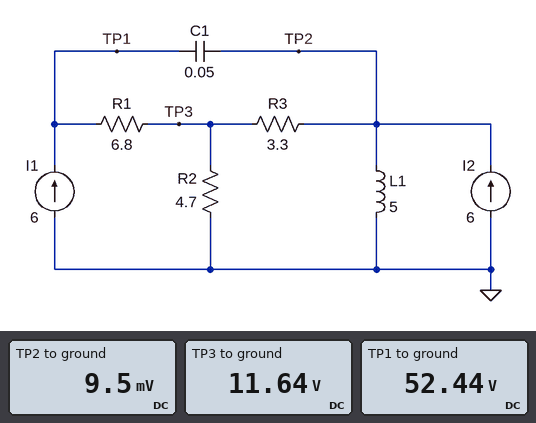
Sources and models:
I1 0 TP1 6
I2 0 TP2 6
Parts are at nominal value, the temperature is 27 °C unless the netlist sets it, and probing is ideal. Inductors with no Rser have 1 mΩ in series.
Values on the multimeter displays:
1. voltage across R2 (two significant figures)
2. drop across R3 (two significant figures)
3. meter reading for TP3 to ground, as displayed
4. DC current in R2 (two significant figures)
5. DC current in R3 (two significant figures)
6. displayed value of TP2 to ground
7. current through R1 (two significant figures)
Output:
12 V
12 V
11.64 V
2.5 A
3.5 A
9.5 mV
6.0 A
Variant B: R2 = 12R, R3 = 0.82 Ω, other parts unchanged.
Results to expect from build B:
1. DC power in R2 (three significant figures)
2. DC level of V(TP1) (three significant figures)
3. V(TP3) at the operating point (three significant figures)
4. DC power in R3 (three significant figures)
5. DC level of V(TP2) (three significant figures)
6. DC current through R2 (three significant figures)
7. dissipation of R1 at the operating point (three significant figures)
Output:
1.78 W
45.4 V
4.62 V
25.9 W
11.6 mV
385 mA
245 W
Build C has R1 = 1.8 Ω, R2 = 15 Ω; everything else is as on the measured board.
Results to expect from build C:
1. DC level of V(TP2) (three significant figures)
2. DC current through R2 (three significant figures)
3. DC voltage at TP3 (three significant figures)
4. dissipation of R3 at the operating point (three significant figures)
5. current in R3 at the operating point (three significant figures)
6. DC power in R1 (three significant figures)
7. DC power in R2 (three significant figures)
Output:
10.9 mV
1.08 A
16.2 V
79.8 W
4.92 A
64.8 W
17.6 W
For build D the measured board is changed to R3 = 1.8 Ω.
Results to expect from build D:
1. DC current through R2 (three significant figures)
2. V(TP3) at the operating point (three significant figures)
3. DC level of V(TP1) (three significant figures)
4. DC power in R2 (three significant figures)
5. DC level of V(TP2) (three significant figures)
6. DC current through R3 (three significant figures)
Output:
1.66 A
7.82 V
48.6 V
13.0 W
10.3 mV
4.34 A
